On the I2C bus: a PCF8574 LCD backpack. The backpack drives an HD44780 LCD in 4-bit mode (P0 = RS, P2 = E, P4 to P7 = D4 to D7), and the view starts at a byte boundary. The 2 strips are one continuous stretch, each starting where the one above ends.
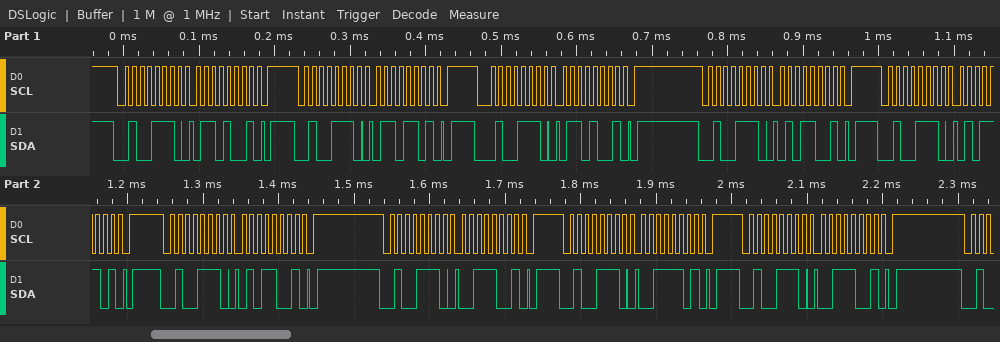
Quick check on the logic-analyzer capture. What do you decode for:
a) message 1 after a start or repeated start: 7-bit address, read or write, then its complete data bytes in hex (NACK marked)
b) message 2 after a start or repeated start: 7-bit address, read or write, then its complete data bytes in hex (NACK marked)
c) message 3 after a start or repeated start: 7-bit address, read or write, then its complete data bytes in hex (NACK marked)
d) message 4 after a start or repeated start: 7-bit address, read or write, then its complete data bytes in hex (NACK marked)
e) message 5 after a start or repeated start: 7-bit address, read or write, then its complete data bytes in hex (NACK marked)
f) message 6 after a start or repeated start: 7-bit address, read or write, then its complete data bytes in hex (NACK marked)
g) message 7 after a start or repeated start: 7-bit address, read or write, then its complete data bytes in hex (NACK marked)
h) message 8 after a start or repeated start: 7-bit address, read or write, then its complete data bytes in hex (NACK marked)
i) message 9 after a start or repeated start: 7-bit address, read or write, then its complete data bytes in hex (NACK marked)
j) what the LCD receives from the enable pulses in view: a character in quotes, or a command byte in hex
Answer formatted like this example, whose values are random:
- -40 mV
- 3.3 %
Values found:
- 0x27 write: 69
- 0x27 write: 6D
- 0x27 write: 69
- 0x27 write: 59
- 0x27 write: 5D
- 0x27 write: 59
- 0x27 write: 39
- 0x27 write: 3D
- 0x27 write: 39
- 'e'
